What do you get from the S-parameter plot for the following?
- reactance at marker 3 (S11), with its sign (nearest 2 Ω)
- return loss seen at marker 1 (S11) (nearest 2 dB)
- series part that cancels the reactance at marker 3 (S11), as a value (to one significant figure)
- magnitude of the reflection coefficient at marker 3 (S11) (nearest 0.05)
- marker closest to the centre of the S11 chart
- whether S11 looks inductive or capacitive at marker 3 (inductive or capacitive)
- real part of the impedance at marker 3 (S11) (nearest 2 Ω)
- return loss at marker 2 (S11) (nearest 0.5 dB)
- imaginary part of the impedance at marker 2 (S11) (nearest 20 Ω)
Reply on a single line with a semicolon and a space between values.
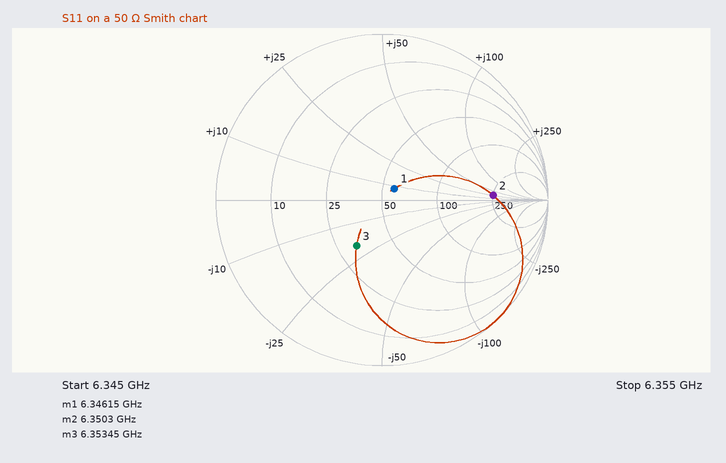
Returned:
-20 Ω; 20 dB; 500 pH; 0.30; marker 1; capacitive; 32 Ω; 3.5 dB; +20 Ω
